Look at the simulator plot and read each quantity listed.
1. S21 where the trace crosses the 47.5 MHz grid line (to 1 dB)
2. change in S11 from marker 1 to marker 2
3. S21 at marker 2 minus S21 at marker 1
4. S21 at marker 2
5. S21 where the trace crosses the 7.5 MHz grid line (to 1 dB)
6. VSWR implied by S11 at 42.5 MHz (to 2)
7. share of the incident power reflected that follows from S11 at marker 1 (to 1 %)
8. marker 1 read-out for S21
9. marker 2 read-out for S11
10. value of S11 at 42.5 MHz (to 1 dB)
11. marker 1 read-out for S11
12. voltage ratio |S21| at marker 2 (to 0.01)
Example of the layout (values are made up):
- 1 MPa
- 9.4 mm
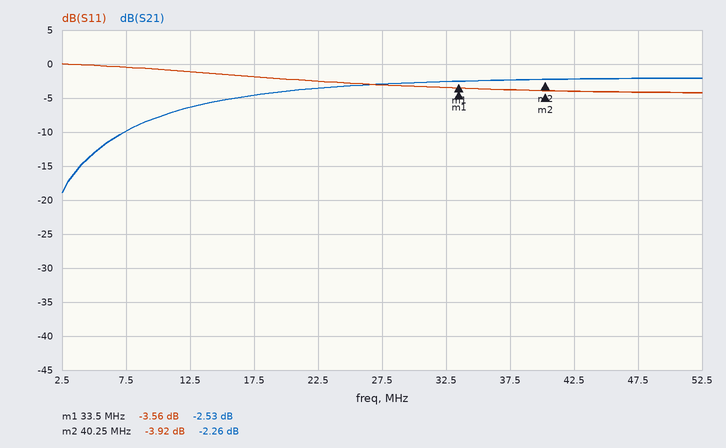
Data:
- -2 dB
- -0.36 dB
- 0.27 dB
- -2.26 dB
- -10 dB
- 4
- 44 %
- -2.53 dB
- -3.92 dB
- -4 dB
- -3.56 dB
- 0.77
